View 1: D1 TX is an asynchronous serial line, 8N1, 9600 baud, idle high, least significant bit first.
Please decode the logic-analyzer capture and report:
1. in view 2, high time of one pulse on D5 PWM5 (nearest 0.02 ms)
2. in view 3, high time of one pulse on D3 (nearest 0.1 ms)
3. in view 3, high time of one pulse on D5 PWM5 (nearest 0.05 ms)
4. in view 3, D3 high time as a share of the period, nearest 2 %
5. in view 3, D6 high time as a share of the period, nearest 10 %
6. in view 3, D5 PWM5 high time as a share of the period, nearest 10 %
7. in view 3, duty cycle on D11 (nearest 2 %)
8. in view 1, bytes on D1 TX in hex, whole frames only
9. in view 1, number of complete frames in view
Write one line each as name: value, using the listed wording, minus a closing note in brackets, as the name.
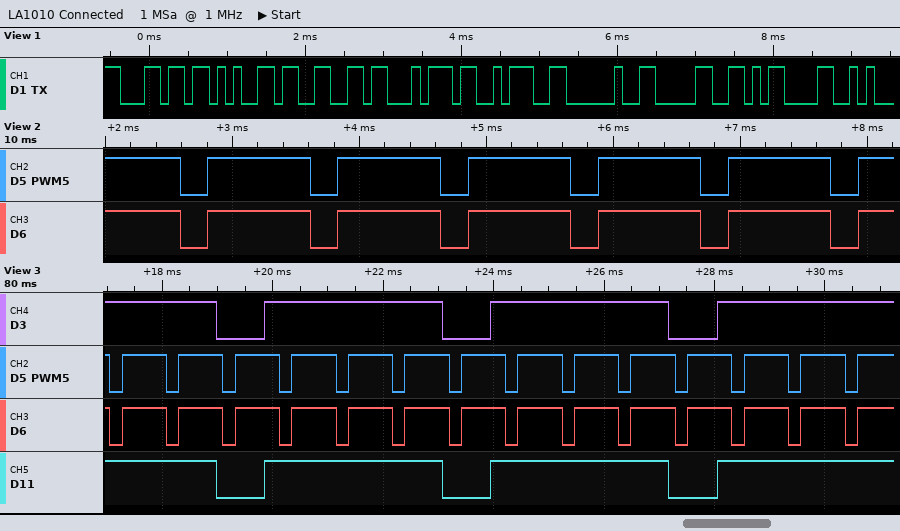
in view 2, high time of one pulse on D5 PWM5: 0.80 ms
in view 3, high time of one pulse on D3: 3.2 ms
in view 3, high time of one pulse on D5 PWM5: 0.80 ms
in view 3, D3 high time as a share of the period, nearest 2 %: 78 %
in view 3, D6 high time as a share of the period, nearest 10 %: 80 %
in view 3, D5 PWM5 high time as a share of the period, nearest 10 %: 80 %
in view 3, duty cycle on D11: 78 %
in view 1, bytes on D1 TX in hex, whole frames only: 6C 65 66 74 3A 20 30 0D
in view 1, number of complete frames in view: 8
